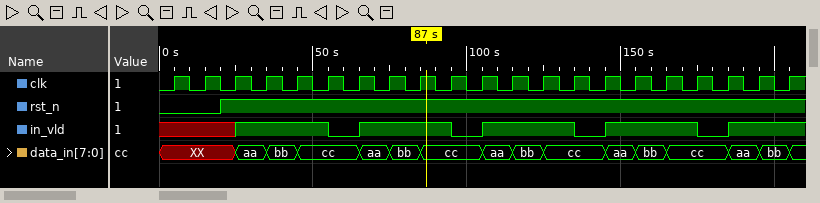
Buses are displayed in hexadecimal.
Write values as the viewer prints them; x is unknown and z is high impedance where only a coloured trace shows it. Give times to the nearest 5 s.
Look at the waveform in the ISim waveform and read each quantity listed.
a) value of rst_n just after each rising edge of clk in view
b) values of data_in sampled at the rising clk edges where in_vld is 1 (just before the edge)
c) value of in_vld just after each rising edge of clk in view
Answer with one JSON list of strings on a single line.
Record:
["0 0 1 1 1 1 1 1 1 1 1 1 1 1 1 1 1 1 1 1 1", "aa, bb, cc, aa, bb, cc, aa, bb, cc, aa, bb, cc, aa, bb", "x x 1 1 1 0 1 1 1 0 1 1 1 0 1 1 1 0 1 1 1"]
